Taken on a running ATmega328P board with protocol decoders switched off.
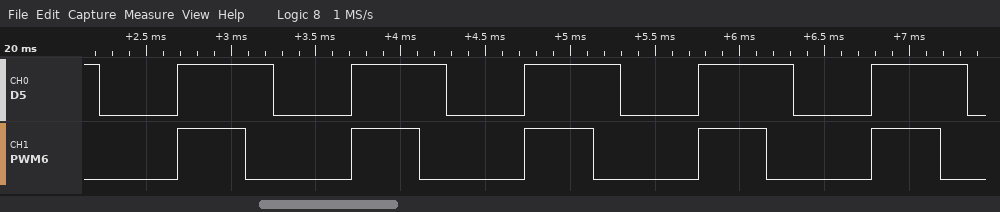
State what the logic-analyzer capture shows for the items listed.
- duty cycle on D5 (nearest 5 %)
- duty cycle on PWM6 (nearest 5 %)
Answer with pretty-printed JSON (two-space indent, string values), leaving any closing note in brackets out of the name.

{
  "duty cycle on D5": "55 %",
  "duty cycle on PWM6": "40 %"
}
